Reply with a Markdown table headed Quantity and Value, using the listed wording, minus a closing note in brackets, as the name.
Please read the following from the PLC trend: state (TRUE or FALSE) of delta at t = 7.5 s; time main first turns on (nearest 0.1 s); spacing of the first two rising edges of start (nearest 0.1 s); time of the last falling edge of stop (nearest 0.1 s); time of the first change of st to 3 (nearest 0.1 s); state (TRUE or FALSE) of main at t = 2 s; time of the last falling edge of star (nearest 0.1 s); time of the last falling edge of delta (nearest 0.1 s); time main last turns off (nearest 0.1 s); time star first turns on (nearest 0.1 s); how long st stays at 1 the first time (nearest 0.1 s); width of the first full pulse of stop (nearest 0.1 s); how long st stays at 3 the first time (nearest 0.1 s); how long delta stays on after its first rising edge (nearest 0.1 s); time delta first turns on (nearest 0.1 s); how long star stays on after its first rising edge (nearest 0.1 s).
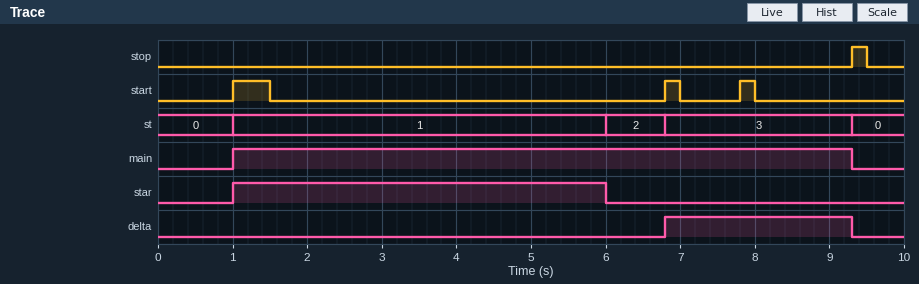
| Quantity | Value |
|---|---|
| state (TRUE or FALSE) of delta at t = 7.5 s | TRUE |
| time main first turns on | 1.0 s |
| spacing of the first two rising edges of start | 5.8 s |
| time of the last falling edge of stop | 9.5 s |
| time of the first change of st to 3 | 6.8 s |
| state (TRUE or FALSE) of main at t = 2 s | TRUE |
| time of the last falling edge of star | 6.0 s |
| time of the last falling edge of delta | 9.3 s |
| time main last turns off | 9.3 s |
| time star first turns on | 1.0 s |
| how long st stays at 1 the first time | 5.0 s |
| width of the first full pulse of stop | 0.2 s |
| how long st stays at 3 the first time | 2.5 s |
| how long delta stays on after its first rising edge | 2.5 s |
| time delta first turns on | 6.8 s |
| how long star stays on after its first rising edge | 5.0 s |
